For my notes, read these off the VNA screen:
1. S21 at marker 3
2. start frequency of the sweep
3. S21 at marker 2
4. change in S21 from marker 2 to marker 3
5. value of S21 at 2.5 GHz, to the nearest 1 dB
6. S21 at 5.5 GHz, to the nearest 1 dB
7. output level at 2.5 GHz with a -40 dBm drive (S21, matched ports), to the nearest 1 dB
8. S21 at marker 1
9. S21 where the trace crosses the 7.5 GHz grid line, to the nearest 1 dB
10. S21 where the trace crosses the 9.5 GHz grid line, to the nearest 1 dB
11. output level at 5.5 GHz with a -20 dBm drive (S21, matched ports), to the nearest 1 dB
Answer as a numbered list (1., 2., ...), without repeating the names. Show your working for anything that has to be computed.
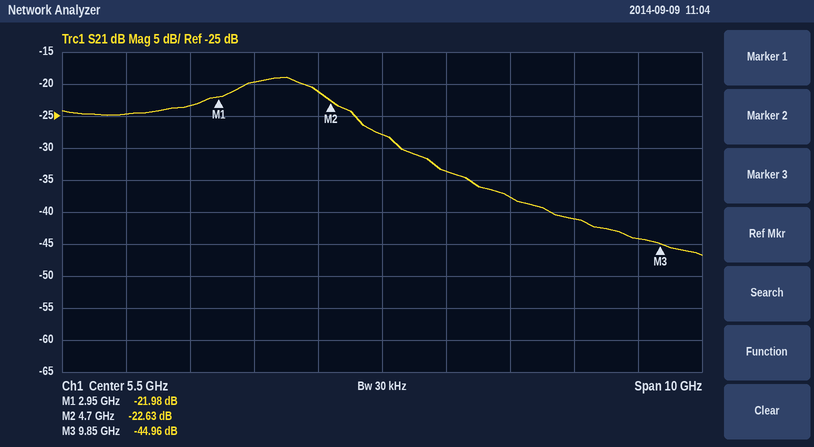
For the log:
1. -44.96 dB
2. 500 MHz
3. -22.63 dB
4. -44.96 − (-22.63) = -22.33 dB
5. -23 dB
6. -28 dB
7. -40 dBm + (-23 dB) = -63 dBm
8. -21.98 dB
9. -38 dB
10. -44 dB
11. -20 dBm + (-28 dB) = -48 dBm
